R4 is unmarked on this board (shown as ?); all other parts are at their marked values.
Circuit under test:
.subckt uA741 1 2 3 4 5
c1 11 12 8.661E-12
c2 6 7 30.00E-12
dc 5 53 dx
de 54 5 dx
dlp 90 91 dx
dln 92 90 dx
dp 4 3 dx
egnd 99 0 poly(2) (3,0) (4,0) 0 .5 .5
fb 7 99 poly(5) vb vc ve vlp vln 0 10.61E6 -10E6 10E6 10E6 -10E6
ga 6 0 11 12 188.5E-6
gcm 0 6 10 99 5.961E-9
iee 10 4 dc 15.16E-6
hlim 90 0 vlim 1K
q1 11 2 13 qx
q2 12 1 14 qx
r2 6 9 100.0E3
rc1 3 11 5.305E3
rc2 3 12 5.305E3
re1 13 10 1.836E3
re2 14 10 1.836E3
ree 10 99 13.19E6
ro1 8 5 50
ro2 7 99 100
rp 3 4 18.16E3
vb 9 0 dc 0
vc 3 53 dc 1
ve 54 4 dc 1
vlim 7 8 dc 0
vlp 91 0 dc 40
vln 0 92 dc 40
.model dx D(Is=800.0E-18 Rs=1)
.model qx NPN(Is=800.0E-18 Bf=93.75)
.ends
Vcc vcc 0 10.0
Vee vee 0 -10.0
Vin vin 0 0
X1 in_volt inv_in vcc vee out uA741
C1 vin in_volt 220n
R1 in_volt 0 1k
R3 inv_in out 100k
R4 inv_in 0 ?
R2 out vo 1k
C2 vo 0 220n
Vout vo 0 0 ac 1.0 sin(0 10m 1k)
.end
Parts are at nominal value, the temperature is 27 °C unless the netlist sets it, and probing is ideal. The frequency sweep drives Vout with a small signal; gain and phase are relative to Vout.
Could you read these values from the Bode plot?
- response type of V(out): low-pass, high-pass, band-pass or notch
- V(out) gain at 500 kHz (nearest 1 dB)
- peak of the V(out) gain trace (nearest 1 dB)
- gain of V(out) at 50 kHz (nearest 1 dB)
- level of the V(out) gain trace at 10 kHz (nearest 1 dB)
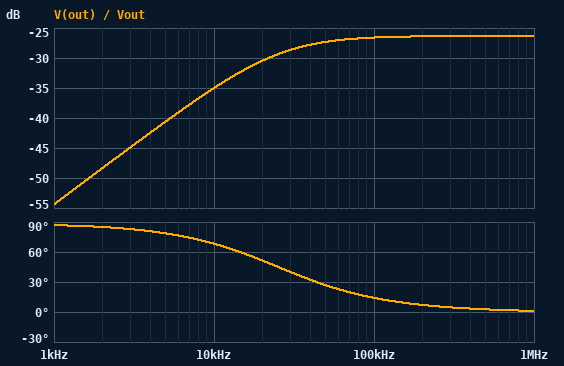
high-pass
-26 dB
-26 dB
-27 dB
-35 dB
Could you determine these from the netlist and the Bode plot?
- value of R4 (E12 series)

2.7 kΩ
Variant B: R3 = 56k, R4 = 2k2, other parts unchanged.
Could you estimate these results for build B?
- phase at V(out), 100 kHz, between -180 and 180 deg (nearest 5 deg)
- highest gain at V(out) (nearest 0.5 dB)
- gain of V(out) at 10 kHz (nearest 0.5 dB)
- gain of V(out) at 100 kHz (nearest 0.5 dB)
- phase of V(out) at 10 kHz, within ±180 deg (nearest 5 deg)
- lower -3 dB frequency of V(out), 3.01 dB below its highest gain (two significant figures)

20 deg
-26.5 dB
-38.0 dB
-27.0 dB
75 deg
36 kHz
